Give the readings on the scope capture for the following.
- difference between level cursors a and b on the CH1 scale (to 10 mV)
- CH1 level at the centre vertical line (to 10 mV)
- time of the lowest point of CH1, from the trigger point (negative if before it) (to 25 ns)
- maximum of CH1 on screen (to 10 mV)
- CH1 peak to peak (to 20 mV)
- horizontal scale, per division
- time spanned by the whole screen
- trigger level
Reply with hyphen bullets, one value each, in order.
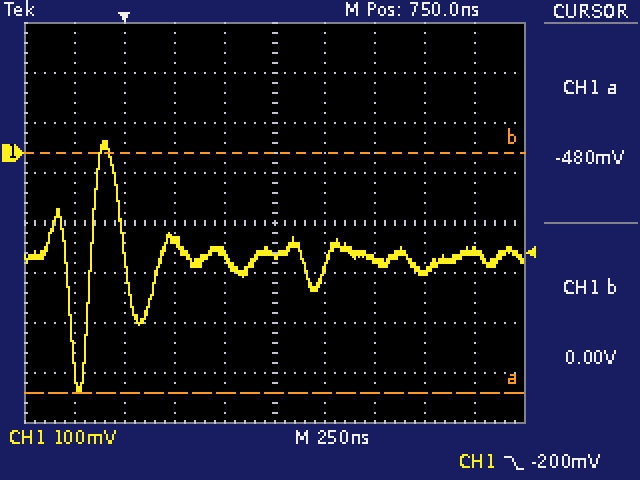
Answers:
- 480 mV
- -200 mV
- -225 ns
- 20 mV
- 500 mV
- 250 ns
- 2.5 µs
- -200 mV
